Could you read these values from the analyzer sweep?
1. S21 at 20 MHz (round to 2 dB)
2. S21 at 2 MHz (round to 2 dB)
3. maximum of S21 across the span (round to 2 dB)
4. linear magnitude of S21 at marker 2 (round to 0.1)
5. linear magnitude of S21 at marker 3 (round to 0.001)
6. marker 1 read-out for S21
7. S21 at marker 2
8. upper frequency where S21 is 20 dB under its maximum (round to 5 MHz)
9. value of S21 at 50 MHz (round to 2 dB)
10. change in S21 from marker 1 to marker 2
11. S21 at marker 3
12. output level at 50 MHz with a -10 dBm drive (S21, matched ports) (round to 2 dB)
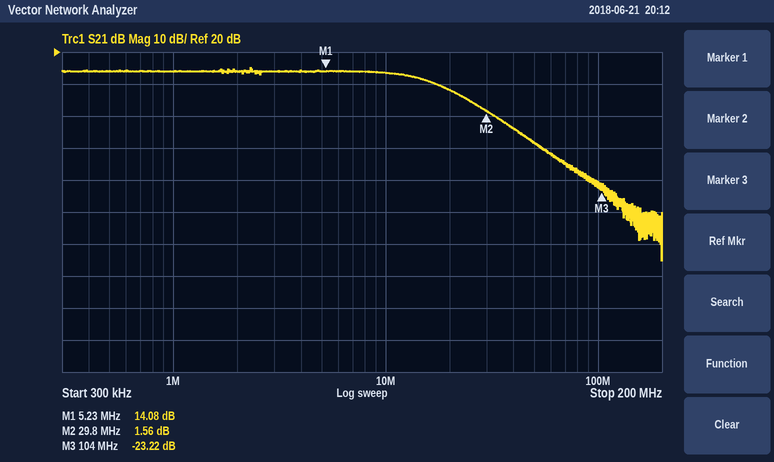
8 dB
14 dB
16 dB
1.2
0.069
14.08 dB
1.56 dB
40 MHz
-8 dB
-12.52 dB
-23.22 dB
-18 dBm
